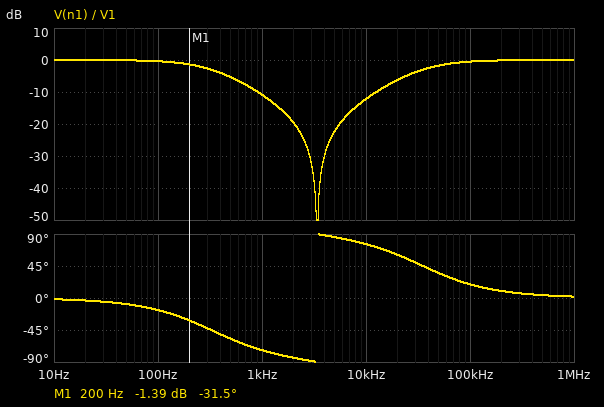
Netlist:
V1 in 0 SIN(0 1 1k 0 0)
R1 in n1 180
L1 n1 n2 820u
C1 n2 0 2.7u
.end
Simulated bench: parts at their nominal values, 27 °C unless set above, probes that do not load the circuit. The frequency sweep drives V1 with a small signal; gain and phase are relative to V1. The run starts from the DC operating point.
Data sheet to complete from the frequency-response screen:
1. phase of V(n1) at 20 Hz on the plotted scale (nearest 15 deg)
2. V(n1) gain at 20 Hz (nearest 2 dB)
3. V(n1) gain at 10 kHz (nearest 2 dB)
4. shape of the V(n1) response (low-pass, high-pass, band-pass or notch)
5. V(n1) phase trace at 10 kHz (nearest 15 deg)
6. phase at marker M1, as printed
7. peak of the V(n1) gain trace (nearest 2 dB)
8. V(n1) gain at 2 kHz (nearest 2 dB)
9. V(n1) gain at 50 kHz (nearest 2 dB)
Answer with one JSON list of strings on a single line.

["0 deg", "0 dB", "-12 dB", "notch", "75 deg", "-31.5 deg", "0 dB", "-20 dB", "-2 dB"]
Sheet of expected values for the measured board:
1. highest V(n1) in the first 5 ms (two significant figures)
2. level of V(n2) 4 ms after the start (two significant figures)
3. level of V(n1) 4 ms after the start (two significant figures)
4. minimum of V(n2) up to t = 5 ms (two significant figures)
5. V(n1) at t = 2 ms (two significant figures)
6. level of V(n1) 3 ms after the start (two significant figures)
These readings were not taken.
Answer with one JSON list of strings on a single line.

["410 mV", "-300 mV", "-270 mV", "-310 mV", "-270 mV", "-270 mV"]
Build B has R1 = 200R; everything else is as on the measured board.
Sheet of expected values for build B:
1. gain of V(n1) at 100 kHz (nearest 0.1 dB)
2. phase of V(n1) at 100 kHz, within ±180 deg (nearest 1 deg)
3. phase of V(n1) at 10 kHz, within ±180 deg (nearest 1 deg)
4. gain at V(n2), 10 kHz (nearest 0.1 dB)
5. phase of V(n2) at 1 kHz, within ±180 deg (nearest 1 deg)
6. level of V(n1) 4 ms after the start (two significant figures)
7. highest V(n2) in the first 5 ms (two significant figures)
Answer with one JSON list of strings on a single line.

["-0.6 dB", "21 deg", "77 deg", "-30.8 dB", "-75 deg", "-250 mV", "400 mV"]
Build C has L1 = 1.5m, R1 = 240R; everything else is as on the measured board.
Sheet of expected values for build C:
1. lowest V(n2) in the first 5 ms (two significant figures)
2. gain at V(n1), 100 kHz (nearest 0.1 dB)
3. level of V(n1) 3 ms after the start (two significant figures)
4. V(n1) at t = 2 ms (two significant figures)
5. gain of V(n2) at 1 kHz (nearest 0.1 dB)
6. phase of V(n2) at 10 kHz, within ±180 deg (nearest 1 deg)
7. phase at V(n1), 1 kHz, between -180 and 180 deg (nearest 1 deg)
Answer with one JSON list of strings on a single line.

["-240 mV", "-0.3 dB", "-200 mV", "-190 mV", "-12.4 dB", "-110 deg", "-78 deg"]
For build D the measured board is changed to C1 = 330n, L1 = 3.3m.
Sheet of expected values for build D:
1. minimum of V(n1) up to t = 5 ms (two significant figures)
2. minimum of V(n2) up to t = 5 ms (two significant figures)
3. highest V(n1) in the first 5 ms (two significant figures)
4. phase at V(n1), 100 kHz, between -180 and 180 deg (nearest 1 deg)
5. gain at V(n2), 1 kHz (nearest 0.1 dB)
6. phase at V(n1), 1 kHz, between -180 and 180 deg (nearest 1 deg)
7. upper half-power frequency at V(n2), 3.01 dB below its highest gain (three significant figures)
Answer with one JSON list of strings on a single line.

["-930 mV", "-970 mV", "930 mV", "5 deg", "-0.2 dB", "-21 deg", "3.60 kHz"]
